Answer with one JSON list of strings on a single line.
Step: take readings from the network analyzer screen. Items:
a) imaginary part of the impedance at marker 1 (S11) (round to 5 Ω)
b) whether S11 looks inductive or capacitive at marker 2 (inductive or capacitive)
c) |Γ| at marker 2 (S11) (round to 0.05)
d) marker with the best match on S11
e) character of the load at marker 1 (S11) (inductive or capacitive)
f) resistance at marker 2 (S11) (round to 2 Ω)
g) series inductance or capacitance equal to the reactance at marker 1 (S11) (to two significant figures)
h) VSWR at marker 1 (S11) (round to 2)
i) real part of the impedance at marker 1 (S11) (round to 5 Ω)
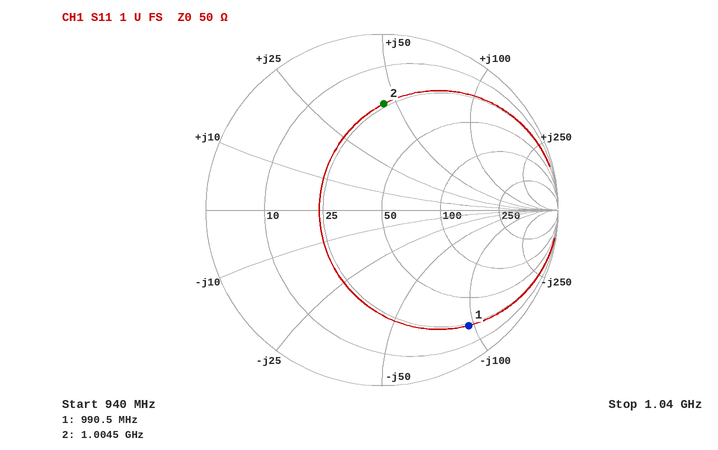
["-95 Ω", "inductive", "0.60", "marker 2", "capacitive", "24 Ω", "1.7 pF", "10", "25 Ω"]
